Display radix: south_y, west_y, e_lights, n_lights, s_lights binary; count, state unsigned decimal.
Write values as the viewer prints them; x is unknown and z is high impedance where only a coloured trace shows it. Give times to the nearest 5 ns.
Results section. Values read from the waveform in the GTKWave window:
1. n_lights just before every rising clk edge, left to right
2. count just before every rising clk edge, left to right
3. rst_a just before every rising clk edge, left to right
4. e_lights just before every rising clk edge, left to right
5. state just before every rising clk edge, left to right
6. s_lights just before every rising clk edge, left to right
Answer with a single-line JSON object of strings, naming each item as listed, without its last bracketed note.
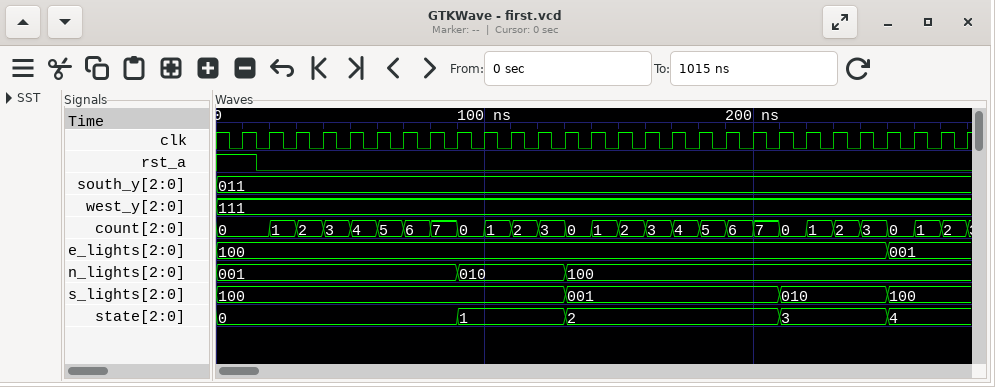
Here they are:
{"n_lights just before every rising clk edge, left to right": "001, 001, 001, 001, 001, 001, 001, 001, 001, 010, 010, 010, 010, 100, 100, 100, 100, 100, 100, 100, 100, 100, 100, 100, 100, 100, 100, 100", "count just before every rising clk edge, left to right": "0, 0, 1, 2, 3, 4, 5, 6, 7, 0, 1, 2, 3, 0, 1, 2, 3, 4, 5, 6, 7, 0, 1, 2, 3, 0, 1, 2", "rst_a just before every rising clk edge, left to right": "1 0 0 0 0 0 0 0 0 0 0 0 0 0 0 0 0 0 0 0 0 0 0 0 0 0 0 0", "e_lights just before every rising clk edge, left to right": "100, 100, 100, 100, 100, 100, 100, 100, 100, 100, 100, 100, 100, 100, 100, 100, 100, 100, 100, 100, 100, 100, 100, 100, 100, 001, 001, 001", "state just before every rising clk edge, left to right": "0, 0, 0, 0, 0, 0, 0, 0, 0, 1, 1, 1, 1, 2, 2, 2, 2, 2, 2, 2, 2, 3, 3, 3, 3, 4, 4, 4", "s_lights just before every rising clk edge, left to right": "100, 100, 100, 100, 100, 100, 100, 100, 100, 100, 100, 100, 100, 001, 001, 001, 001, 001, 001, 001, 001, 010, 010, 010, 010, 100, 100, 100"}
